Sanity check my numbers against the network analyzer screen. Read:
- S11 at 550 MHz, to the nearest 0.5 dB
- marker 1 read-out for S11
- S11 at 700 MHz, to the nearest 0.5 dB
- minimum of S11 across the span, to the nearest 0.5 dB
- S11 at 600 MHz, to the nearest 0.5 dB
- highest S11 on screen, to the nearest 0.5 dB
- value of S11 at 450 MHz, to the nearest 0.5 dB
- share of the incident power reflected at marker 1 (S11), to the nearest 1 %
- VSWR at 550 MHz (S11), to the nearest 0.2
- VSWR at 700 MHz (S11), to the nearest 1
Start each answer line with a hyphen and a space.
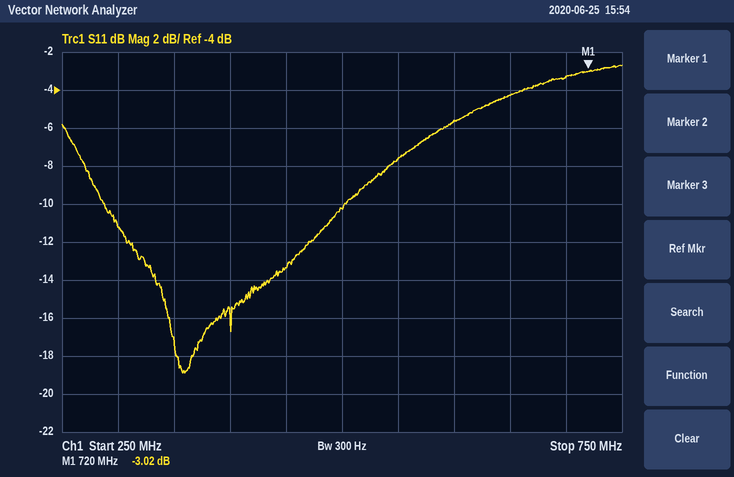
- -7.5 dB
- -3.02 dB
- -3.5 dB
- -19.0 dB
- -5.5 dB
- -2.5 dB
- -13.5 dB
- 50 %
- 2.4
- 5
